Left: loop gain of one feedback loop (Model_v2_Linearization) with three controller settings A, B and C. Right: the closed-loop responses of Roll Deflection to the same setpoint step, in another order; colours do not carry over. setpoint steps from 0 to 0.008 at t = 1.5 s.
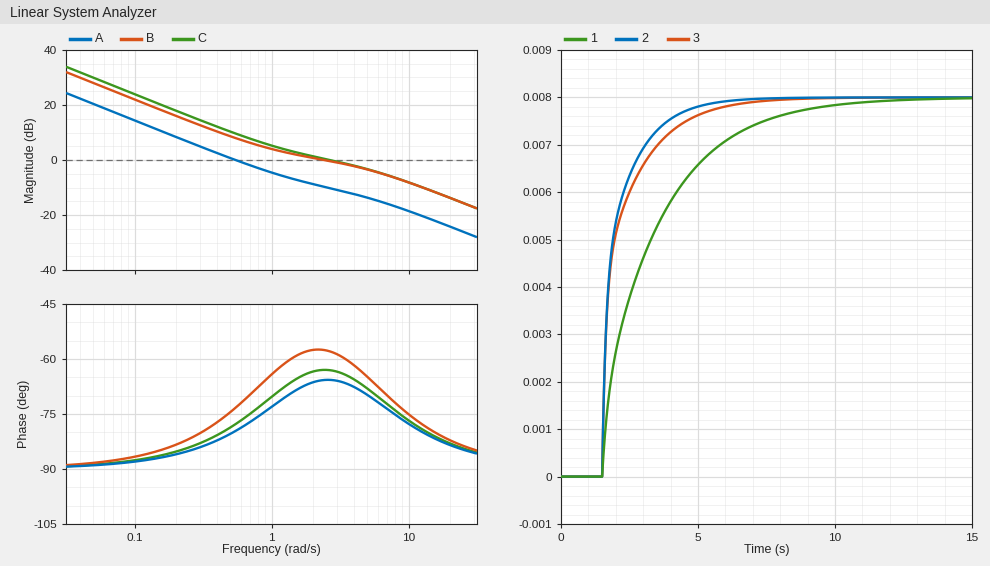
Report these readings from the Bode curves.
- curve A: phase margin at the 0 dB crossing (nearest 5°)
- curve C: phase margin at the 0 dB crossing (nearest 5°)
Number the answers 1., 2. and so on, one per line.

1. 100°
2. 115°
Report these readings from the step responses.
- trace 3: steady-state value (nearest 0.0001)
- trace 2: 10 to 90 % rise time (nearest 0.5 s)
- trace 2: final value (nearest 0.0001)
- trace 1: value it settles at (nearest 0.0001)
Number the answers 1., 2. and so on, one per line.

1. 0.0080
2. 2.0 s
3. 0.0080
4. 0.0080
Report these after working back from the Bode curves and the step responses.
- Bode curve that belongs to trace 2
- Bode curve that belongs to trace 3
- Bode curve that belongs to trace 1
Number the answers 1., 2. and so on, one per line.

1. C
2. B
3. A
